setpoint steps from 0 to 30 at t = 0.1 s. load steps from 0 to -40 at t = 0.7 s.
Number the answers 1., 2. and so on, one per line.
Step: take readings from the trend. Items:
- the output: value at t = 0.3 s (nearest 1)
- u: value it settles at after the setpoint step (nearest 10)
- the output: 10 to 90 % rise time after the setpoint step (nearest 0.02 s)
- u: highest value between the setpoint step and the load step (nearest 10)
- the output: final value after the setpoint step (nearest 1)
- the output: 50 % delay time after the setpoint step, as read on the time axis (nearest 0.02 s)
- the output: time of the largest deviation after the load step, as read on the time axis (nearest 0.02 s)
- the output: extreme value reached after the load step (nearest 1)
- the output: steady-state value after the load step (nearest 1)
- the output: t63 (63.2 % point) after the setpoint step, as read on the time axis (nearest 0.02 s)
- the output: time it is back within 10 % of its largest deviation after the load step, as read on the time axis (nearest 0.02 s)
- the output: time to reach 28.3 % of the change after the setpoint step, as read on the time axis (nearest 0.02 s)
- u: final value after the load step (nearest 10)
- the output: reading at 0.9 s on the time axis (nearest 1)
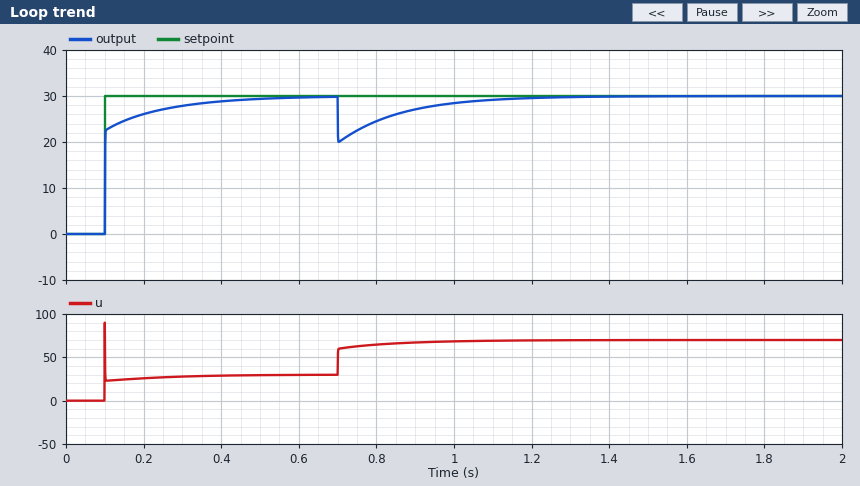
1. 28
2. 30
3. 0.14 s
4. 90
5. 30
6. 0.10 s
7. 0.70 s
8. 20
9. 30
10. 0.10 s
11. 1.08 s
12. 0.10 s
13. 70
14. 27
